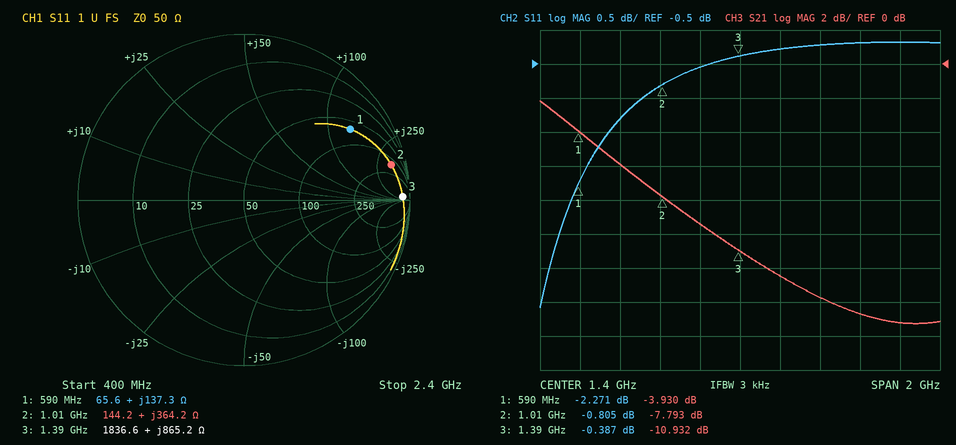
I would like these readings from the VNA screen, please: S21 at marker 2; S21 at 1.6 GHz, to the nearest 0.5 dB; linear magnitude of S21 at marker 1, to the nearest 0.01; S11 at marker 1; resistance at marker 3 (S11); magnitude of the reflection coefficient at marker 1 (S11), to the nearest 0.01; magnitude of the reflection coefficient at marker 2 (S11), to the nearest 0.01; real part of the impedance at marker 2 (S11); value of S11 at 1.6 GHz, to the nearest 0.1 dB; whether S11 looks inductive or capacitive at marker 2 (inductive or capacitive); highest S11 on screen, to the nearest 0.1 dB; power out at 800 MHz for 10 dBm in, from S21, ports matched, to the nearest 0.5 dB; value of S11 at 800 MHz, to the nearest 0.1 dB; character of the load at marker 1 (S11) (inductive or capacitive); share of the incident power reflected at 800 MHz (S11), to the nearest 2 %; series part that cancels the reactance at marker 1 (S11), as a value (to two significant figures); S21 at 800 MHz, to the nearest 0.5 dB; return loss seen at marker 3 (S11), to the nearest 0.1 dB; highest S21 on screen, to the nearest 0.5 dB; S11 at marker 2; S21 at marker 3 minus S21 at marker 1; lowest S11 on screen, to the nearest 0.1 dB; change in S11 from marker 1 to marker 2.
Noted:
-7.793 dB
-12.5 dB
0.64
-2.271 dB
1836.6 Ω
0.77
0.91
144.2 Ω
-0.3 dB
inductive
-0.2 dB
4.0 dBm
-1.3 dB
inductive
74 %
2.0 pF
-6.0 dB
0.4 dB
-2.0 dB
-0.805 dB
-7.002 dB
-4.1 dB
1.466 dB
